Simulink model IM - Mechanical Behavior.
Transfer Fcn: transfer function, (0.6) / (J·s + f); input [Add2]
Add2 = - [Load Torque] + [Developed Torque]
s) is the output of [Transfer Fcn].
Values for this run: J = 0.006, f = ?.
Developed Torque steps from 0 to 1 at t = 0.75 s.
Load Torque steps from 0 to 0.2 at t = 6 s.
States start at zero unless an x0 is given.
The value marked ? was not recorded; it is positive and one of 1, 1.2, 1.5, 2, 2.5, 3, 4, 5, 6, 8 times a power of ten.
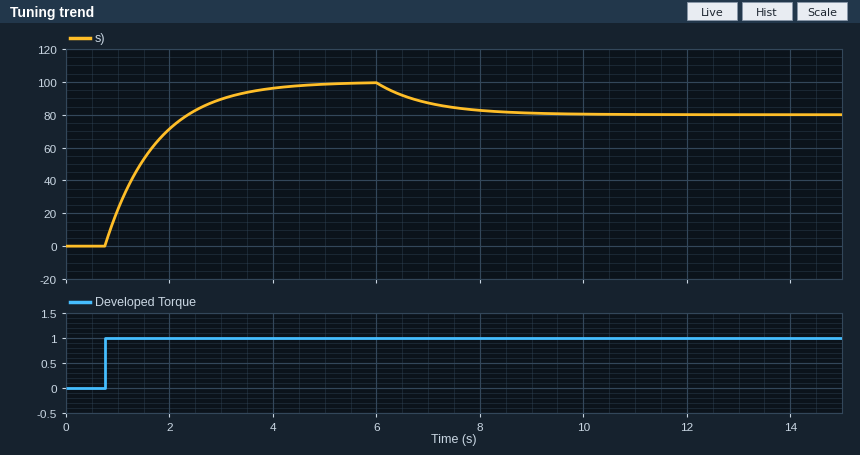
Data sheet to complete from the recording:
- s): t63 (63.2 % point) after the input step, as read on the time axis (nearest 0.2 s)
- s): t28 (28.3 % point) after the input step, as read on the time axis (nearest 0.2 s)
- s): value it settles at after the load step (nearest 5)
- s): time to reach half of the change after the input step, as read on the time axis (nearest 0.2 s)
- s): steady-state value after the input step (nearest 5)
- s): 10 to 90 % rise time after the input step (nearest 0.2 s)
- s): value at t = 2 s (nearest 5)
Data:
1.8 s
1.0 s
80
1.4 s
100
2.2 s
70
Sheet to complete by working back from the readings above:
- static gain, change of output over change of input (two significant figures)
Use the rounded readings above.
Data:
100
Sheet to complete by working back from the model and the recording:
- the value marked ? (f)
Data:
0.006
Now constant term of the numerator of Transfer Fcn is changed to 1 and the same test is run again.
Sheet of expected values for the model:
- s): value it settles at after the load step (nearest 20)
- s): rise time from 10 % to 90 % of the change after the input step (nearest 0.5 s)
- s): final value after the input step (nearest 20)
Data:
140
2.0 s
160
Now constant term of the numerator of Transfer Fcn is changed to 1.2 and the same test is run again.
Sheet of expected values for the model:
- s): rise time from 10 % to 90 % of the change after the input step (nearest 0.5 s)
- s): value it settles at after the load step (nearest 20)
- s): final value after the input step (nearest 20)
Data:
2.0 s
160
200
